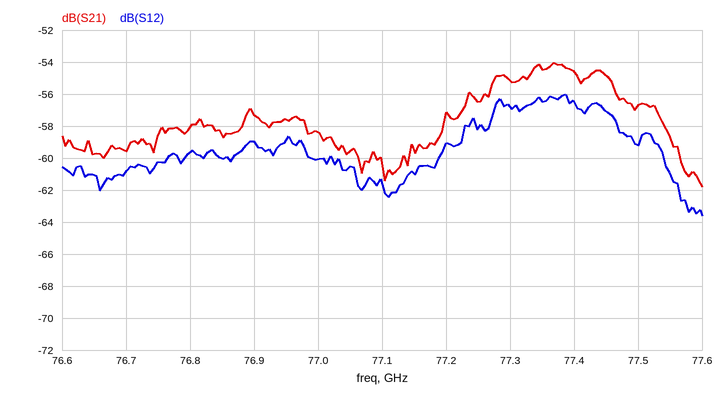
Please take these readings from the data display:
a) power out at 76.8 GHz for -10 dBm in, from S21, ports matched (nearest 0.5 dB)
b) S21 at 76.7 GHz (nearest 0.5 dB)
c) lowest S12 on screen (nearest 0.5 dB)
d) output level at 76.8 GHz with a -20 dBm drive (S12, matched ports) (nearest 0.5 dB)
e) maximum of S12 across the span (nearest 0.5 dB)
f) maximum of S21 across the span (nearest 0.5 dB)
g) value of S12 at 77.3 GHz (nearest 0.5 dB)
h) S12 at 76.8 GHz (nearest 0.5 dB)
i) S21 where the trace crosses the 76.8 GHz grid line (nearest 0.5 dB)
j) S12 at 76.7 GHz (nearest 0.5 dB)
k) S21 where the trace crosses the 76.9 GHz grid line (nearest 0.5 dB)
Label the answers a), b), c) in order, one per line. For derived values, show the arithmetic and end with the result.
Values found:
a) -10 dBm + (-58.0 dB) = -68.0 dBm
b) -59.5 dB
c) -63.5 dB
d) -20 dBm + (-59.5 dB) = -79.5 dBm
e) -56.0 dB
f) -54.0 dB
g) -57.0 dB
h) -59.5 dB
i) -58.0 dB
j) -61.0 dB
k) -57.5 dB
